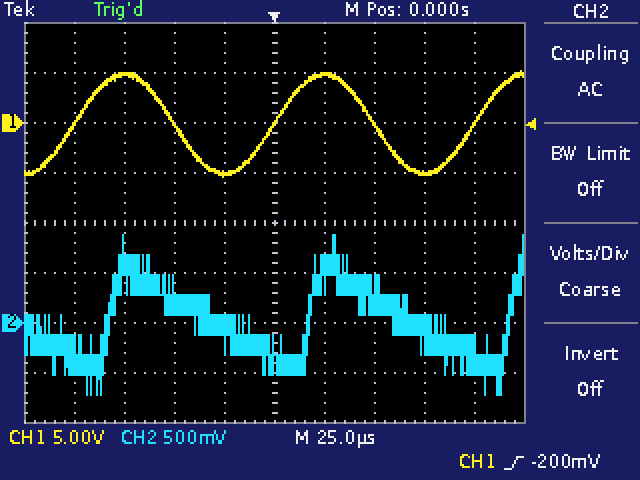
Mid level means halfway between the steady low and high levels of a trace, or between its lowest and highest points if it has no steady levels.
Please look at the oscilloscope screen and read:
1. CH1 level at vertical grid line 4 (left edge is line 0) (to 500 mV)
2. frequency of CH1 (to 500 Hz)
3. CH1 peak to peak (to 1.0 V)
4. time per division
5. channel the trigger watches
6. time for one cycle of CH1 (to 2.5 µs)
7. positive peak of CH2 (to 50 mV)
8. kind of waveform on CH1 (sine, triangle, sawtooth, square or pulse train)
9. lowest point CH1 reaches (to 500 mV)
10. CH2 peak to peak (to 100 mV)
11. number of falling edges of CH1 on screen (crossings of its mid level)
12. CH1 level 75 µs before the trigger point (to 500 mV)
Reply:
-5.0 V
10.0 kHz
11.0 V
25 µs
CH1
100.0 µs
900 mV
sine
-5.5 V
1.60 V
2
5.0 V
